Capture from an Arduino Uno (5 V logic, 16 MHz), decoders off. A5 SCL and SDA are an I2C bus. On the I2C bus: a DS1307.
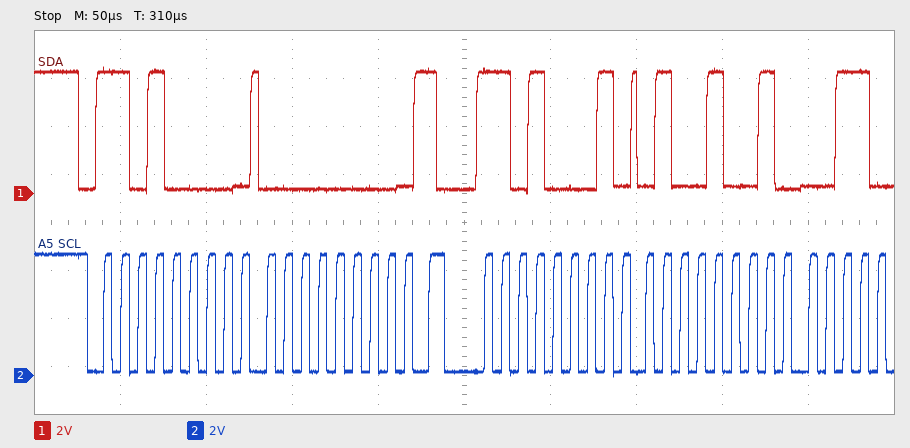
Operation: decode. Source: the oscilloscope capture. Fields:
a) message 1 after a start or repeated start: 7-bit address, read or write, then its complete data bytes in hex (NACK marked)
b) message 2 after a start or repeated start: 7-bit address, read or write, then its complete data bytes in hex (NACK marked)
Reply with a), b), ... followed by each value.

a) 0x68 write: 00
b) 0x68 read: 49
